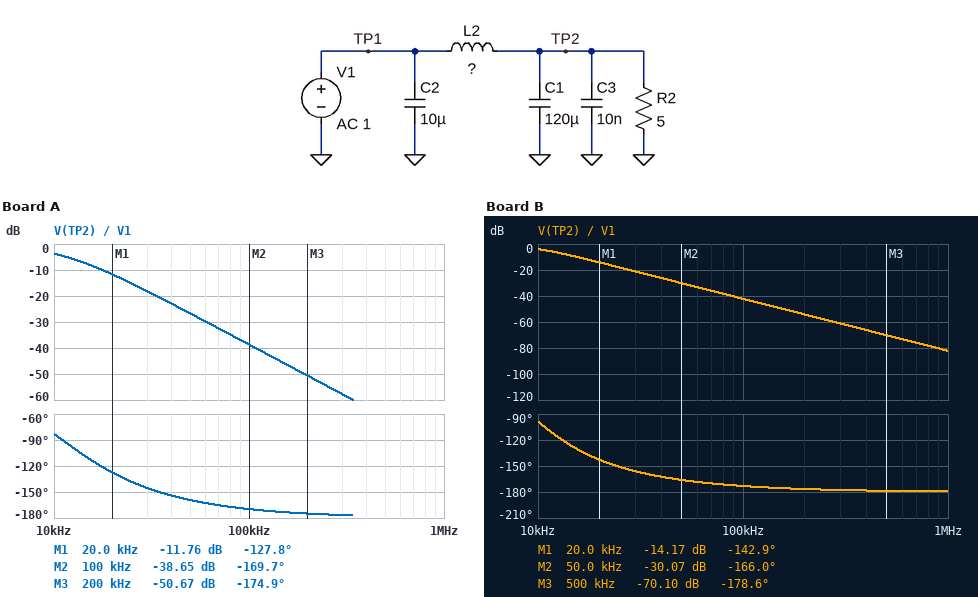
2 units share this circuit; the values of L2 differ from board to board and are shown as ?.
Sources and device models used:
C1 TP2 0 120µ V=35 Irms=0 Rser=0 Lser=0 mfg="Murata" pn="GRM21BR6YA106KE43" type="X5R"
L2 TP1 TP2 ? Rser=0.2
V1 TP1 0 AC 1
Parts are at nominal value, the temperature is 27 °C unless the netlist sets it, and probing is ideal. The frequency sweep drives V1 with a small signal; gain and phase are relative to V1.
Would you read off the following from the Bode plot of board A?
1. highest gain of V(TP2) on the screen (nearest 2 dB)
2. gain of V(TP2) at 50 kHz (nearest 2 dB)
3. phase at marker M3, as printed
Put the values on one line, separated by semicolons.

-4 dB; -26 dB; -174.9 deg
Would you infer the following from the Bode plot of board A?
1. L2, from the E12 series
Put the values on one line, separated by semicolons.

1.8 µH
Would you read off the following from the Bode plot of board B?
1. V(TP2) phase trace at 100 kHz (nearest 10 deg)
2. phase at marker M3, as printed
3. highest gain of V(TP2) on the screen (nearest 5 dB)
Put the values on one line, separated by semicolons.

-170 deg; -178.6 deg; -5 dB
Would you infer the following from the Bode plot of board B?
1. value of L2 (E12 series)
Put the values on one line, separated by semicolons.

2.7 µH
